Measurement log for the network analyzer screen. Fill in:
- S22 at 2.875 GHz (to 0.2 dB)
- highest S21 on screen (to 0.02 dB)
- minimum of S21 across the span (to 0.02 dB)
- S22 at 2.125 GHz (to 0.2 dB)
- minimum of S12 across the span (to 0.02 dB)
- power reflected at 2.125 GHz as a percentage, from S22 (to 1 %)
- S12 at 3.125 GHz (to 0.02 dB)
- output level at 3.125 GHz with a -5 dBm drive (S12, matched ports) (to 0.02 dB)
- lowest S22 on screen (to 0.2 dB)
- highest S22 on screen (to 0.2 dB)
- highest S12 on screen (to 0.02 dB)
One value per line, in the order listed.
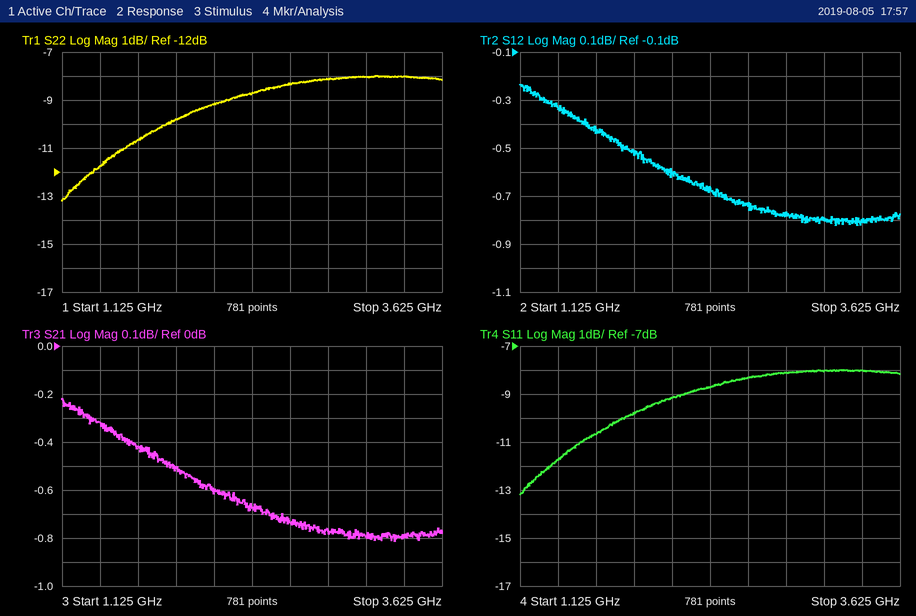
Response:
-8.2 dB
-0.22 dB
-0.82 dB
-9.2 dB
-0.82 dB
12 %
-0.80 dB
-5.80 dBm
-13.2 dB
-8.0 dB
-0.24 dB
